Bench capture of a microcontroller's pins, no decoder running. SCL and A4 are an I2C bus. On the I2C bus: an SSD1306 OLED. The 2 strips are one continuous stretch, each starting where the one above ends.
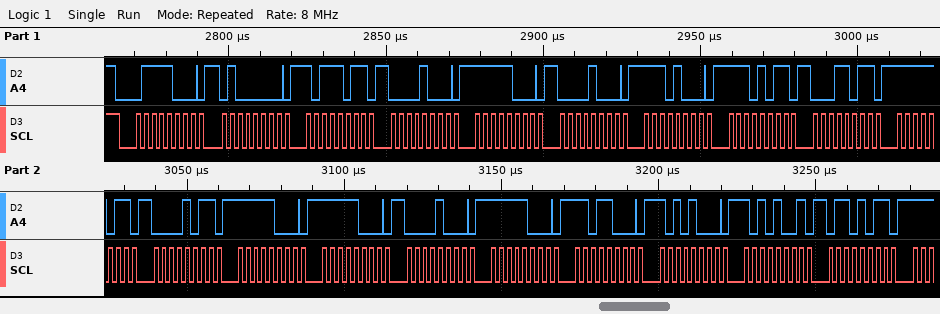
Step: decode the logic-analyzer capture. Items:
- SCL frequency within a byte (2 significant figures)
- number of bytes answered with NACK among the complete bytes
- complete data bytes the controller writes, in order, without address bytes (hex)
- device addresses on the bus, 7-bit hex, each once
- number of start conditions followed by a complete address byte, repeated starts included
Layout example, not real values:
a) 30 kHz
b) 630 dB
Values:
a) 400 kHz
b) 0
c) 40 BB 08 F8 08 E8 EB 1B FB 0B F8 F8 08 F8 D8 A8 A9 6B
d) 0x3C
e) 1
